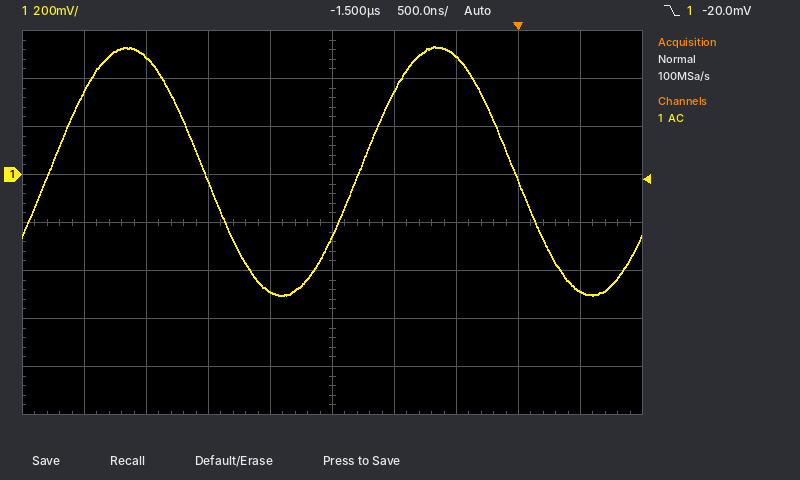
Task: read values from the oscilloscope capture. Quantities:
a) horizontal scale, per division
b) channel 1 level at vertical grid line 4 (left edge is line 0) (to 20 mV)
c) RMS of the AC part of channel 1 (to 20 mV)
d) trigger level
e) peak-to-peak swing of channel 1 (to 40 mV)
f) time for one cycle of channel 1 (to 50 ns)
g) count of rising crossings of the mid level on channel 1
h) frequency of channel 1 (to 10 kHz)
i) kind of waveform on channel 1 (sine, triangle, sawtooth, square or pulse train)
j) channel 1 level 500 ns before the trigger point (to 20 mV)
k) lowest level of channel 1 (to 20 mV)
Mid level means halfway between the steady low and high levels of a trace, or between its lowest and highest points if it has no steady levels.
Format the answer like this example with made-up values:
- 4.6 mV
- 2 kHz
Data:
- 500 ns
- -480 mV
- 360 mV
- -20.0 mV
- 1.04 V
- 2.50 µs
- 2
- 400 kHz
- sine
- 500 mV
- -500 mV
